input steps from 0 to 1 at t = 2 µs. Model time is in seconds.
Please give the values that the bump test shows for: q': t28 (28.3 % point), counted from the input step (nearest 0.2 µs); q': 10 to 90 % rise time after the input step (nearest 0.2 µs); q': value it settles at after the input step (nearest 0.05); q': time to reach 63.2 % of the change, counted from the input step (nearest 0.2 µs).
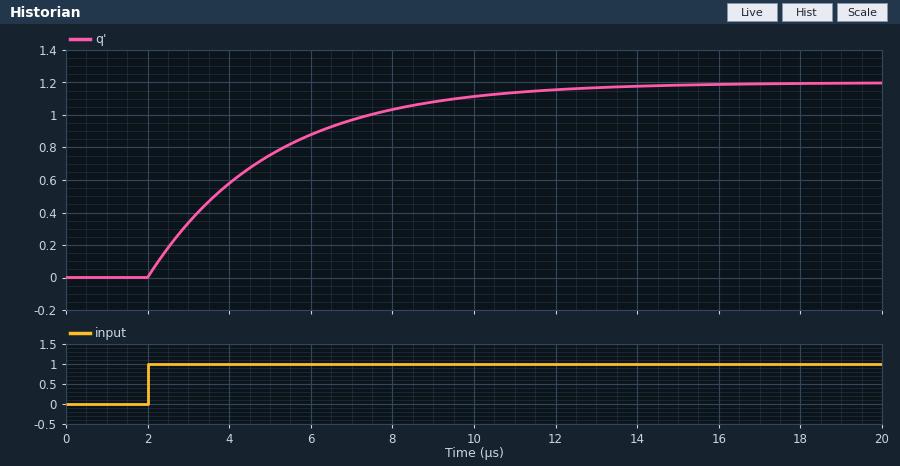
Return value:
1.0 µs
6.6 µs
1.20
3.0 µs
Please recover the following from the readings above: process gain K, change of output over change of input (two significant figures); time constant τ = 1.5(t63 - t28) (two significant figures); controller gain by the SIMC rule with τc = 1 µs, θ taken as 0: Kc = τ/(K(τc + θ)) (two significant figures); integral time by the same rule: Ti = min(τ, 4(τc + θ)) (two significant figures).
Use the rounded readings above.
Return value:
1.2
3.0 µs
2.5
3.0 µs
